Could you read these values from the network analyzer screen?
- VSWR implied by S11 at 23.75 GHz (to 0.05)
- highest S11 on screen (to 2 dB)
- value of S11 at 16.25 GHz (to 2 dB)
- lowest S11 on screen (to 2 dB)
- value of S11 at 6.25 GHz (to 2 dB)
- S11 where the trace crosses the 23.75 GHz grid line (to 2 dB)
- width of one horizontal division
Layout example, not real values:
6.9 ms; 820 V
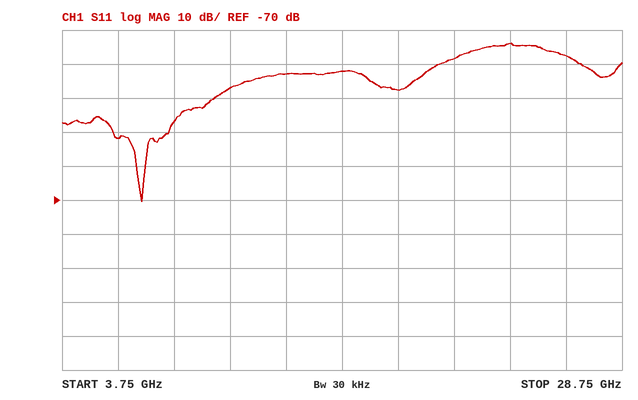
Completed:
1.15; -24 dB; -32 dB; -70 dB; -52 dB; -24 dB; 2.5 GHz
